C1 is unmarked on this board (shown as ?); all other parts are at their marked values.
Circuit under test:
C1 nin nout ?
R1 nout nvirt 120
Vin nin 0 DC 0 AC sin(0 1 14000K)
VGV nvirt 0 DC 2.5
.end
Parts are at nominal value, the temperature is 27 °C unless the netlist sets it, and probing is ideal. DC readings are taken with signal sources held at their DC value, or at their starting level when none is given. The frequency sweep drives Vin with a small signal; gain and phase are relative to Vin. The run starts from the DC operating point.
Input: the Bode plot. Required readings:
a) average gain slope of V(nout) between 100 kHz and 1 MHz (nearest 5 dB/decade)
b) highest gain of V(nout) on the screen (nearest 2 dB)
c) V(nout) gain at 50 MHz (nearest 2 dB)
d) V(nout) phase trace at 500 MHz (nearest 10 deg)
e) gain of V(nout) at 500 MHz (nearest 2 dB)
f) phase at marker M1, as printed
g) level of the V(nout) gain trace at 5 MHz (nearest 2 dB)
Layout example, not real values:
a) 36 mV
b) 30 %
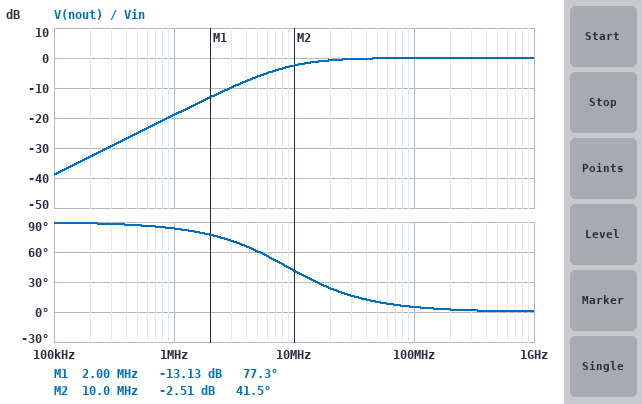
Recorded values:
a) 20 dB/decade
b) 0 dB
c) 0 dB
d) 0 deg
e) 0 dB
f) 77.3 deg
g) -6 dB
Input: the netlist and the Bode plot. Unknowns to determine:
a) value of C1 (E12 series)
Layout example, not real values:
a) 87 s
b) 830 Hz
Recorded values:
a) 150 pF
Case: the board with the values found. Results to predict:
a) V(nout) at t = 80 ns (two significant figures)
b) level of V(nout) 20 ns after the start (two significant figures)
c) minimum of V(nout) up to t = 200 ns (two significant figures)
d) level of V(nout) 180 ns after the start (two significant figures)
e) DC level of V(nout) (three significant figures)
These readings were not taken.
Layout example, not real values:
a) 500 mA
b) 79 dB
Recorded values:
a) 3.3 V
b) 3.0 V
c) 1.6 V
d) 2.0 V
e) 2.50 V
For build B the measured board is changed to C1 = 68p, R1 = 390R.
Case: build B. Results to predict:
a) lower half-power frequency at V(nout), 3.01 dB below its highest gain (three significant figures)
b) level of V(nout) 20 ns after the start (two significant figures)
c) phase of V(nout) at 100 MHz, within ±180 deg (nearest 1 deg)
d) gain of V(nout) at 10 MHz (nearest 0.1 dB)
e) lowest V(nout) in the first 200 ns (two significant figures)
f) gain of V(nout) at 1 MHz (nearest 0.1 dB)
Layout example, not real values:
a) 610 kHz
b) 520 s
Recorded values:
a) 6.00 MHz
b) 3.1 V
c) 3 deg
d) -1.3 dB
e) 1.5 V
f) -15.7 dB
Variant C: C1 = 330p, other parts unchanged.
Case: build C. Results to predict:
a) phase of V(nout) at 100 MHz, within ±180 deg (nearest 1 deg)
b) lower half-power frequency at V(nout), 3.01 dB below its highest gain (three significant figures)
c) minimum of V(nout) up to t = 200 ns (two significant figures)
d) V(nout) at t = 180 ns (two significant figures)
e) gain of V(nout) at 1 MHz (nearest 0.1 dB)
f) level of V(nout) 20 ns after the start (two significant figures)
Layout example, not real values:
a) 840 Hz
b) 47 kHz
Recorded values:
a) 2 deg
b) 4.02 MHz
c) 1.5 V
d) 2.1 V
e) -12.3 dB
f) 3.2 V
